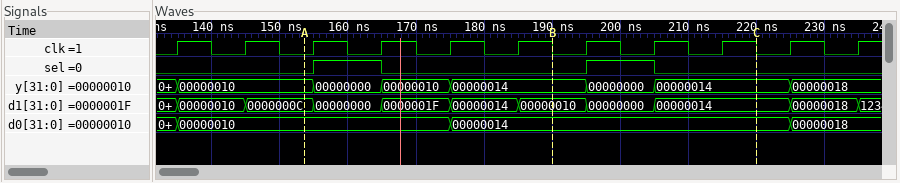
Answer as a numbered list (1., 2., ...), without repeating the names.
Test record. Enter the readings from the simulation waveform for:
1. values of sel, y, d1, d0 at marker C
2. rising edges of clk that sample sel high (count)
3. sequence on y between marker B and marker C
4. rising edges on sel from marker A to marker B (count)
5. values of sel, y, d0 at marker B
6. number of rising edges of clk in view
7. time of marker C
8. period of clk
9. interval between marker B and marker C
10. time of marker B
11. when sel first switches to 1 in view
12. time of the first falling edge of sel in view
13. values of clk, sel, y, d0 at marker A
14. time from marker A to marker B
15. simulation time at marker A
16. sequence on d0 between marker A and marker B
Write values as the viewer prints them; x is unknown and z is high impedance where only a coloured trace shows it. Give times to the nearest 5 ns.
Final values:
1. sel=0, y=00000014, d1=00000014, d0=00000014
2. 2
3. 00000014, 00000000, 00000014
4. 1
5. sel=0, y=00000014, d0=00000014
6. 11
7. 220 ns
8. 10 ns
9. 30 ns
10. 190 ns
11. 155 ns
12. 165 ns
13. clk=0, sel=0, y=00000010, d0=00000010
14. 35 ns
15. 155 ns
16. 00000010, 00000014
